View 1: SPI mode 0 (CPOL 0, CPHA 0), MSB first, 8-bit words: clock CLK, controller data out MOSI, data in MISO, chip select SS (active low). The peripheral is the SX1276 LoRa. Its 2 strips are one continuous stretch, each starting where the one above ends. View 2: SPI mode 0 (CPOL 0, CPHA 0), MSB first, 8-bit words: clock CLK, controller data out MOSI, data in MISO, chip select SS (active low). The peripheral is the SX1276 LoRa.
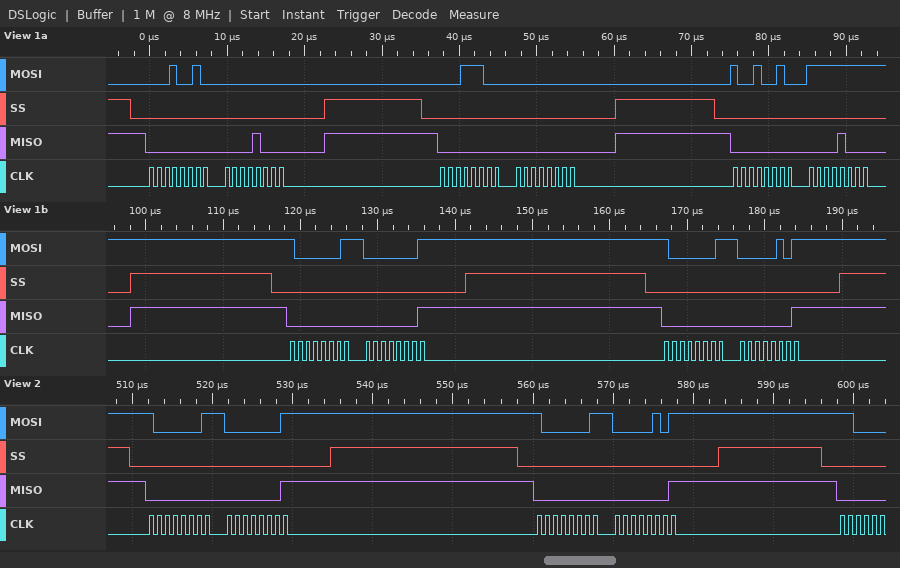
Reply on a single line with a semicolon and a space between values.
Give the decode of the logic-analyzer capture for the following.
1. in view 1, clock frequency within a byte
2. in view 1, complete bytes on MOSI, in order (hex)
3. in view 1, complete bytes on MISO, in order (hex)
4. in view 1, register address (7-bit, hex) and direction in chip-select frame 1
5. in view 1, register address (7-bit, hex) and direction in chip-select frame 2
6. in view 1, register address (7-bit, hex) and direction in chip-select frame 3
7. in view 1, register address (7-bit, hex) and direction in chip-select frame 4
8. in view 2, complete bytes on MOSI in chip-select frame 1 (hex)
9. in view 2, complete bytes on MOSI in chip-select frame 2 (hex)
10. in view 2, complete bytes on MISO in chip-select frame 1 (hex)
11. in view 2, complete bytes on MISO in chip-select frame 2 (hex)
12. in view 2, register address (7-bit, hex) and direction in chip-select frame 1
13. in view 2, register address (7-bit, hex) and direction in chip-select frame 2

1 MHz; 0x12 0x00 0x1C 0x00 0x92 0xFF 0x81 0x01 0x81 0x05; 0x00 0x08 0x00 0x00 0x00 0x08 0x00 0x01 0x00 0x01; 0x12 read; 0x1C read; 0x12 write; 0x01 write; 81 01; 81 05; 00 01; 00 01; 0x01 write; 0x01 write
